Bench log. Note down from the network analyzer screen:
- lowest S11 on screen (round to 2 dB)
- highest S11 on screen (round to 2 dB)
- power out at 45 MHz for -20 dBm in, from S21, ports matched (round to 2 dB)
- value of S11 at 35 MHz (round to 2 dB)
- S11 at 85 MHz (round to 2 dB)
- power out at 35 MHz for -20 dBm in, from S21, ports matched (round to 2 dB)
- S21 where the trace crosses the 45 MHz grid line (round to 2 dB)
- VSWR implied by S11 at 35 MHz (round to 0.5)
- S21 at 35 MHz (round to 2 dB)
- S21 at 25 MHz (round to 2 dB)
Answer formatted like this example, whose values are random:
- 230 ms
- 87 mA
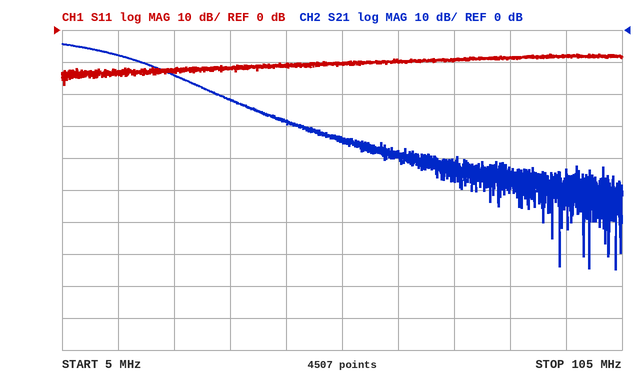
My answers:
- -18 dB
- -8 dB
- -48 dBm
- -12 dB
- -8 dB
- -42 dBm
- -28 dB
- 1.5
- -22 dB
- -14 dB
